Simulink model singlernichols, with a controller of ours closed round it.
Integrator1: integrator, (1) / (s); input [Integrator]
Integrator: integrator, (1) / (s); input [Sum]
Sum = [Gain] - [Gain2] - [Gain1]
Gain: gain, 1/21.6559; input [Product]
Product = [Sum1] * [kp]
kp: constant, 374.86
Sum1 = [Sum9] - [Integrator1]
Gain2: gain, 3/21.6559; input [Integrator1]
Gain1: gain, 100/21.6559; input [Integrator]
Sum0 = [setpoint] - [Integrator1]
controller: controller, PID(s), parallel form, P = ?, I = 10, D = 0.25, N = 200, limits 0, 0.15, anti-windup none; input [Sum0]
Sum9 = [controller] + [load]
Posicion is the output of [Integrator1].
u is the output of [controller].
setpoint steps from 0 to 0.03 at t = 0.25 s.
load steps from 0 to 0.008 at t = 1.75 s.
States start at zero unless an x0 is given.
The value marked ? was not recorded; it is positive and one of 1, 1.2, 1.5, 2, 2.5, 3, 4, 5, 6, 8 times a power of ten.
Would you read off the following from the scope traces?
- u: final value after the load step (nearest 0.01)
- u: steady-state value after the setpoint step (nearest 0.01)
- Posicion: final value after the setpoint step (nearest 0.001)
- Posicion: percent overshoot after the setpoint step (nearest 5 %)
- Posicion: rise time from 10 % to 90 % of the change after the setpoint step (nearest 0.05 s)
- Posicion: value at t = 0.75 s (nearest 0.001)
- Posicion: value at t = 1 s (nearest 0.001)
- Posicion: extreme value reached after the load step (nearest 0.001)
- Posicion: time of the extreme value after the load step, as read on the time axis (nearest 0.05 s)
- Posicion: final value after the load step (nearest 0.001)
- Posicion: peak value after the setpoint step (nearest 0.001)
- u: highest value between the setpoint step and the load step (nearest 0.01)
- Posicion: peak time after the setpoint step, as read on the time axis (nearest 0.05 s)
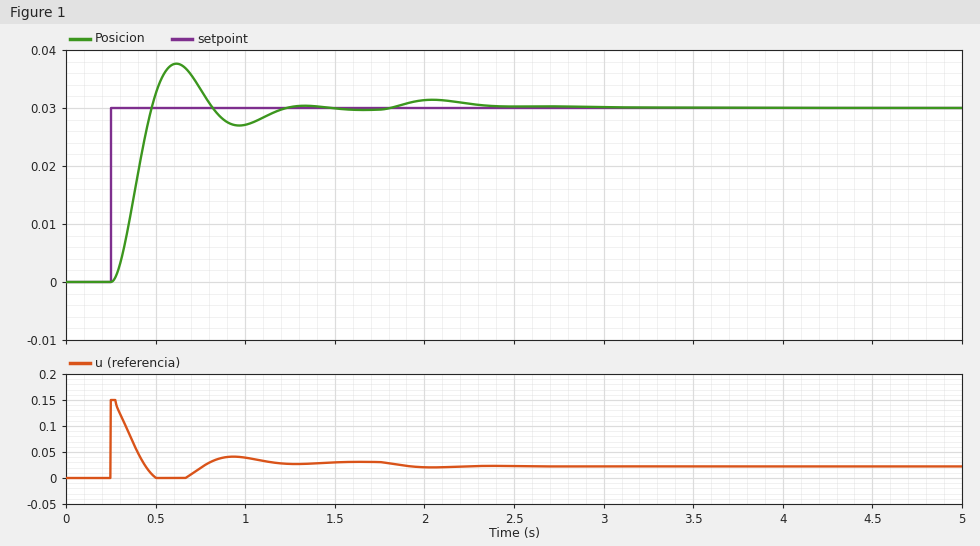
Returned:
0.02
0.03
0.030
25 %
0.15 s
0.033
0.027
0.031
2.05 s
0.030
0.038
0.15
0.60 s
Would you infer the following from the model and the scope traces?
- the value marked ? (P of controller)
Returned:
5
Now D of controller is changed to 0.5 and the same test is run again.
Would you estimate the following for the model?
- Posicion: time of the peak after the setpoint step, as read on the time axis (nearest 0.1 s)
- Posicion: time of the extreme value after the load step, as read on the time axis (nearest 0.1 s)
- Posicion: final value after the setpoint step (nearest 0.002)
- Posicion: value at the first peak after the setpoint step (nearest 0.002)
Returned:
0.7 s
2.1 s
0.030
0.034
